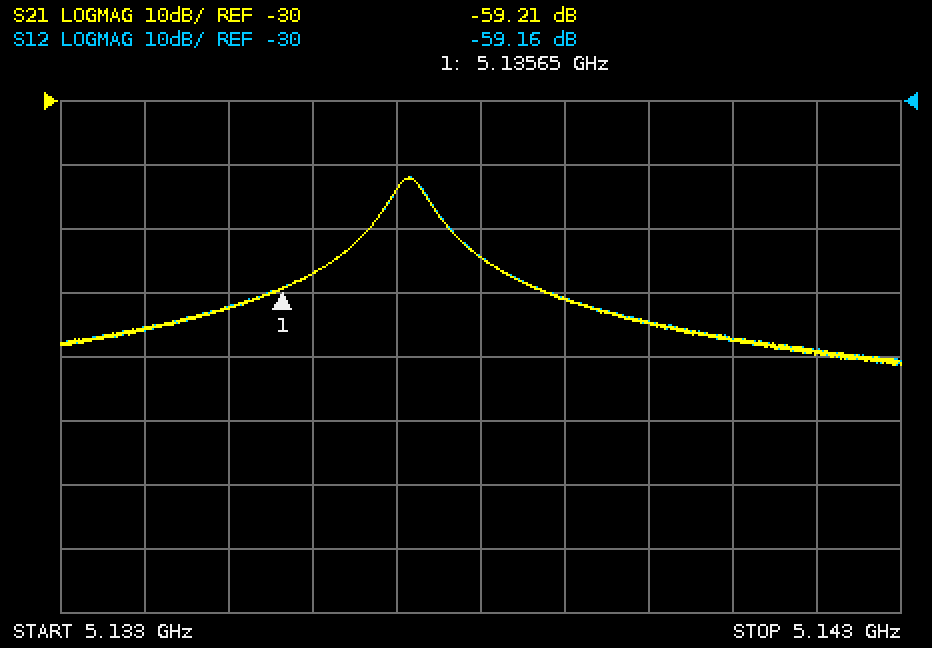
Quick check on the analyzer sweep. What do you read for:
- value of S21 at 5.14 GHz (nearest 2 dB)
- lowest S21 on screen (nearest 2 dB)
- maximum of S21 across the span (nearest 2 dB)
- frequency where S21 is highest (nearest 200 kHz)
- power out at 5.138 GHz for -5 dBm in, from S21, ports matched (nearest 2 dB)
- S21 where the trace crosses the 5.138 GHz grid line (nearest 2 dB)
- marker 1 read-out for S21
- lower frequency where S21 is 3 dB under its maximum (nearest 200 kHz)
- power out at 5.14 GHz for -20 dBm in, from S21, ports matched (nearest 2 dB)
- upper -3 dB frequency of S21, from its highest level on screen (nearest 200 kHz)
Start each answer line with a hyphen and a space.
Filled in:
- -64 dB
- -72 dB
- -42 dB
- 5.1372 GHz
- -60 dBm
- -54 dB
- -59.21 dB
- 5.1370 GHz
- -84 dBm
- 5.1374 GHz
